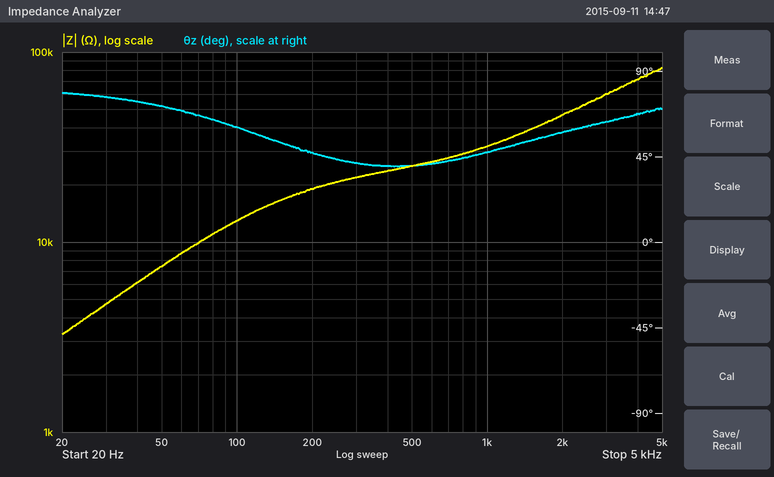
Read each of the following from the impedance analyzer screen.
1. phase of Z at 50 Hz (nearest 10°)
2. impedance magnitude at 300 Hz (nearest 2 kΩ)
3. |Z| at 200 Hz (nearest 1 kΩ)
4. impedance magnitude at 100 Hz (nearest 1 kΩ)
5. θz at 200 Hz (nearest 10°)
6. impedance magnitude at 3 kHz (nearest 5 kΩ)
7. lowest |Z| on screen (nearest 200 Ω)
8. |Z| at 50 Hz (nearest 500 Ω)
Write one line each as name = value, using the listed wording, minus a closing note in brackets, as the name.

phase of Z at 50 Hz = 70°
impedance magnitude at 300 Hz = 22 kΩ
|Z| at 200 Hz = 19 kΩ
impedance magnitude at 100 Hz = 13 kΩ
θz at 200 Hz = 50°
impedance magnitude at 3 kHz = 60 kΩ
lowest |Z| on screen = 3.2 kΩ
|Z| at 50 Hz = 7.5 kΩ
